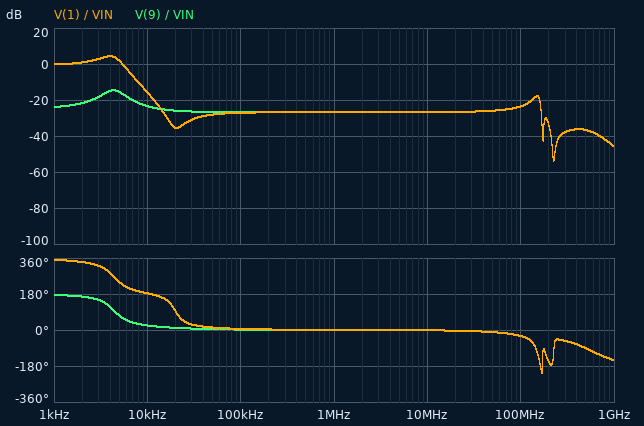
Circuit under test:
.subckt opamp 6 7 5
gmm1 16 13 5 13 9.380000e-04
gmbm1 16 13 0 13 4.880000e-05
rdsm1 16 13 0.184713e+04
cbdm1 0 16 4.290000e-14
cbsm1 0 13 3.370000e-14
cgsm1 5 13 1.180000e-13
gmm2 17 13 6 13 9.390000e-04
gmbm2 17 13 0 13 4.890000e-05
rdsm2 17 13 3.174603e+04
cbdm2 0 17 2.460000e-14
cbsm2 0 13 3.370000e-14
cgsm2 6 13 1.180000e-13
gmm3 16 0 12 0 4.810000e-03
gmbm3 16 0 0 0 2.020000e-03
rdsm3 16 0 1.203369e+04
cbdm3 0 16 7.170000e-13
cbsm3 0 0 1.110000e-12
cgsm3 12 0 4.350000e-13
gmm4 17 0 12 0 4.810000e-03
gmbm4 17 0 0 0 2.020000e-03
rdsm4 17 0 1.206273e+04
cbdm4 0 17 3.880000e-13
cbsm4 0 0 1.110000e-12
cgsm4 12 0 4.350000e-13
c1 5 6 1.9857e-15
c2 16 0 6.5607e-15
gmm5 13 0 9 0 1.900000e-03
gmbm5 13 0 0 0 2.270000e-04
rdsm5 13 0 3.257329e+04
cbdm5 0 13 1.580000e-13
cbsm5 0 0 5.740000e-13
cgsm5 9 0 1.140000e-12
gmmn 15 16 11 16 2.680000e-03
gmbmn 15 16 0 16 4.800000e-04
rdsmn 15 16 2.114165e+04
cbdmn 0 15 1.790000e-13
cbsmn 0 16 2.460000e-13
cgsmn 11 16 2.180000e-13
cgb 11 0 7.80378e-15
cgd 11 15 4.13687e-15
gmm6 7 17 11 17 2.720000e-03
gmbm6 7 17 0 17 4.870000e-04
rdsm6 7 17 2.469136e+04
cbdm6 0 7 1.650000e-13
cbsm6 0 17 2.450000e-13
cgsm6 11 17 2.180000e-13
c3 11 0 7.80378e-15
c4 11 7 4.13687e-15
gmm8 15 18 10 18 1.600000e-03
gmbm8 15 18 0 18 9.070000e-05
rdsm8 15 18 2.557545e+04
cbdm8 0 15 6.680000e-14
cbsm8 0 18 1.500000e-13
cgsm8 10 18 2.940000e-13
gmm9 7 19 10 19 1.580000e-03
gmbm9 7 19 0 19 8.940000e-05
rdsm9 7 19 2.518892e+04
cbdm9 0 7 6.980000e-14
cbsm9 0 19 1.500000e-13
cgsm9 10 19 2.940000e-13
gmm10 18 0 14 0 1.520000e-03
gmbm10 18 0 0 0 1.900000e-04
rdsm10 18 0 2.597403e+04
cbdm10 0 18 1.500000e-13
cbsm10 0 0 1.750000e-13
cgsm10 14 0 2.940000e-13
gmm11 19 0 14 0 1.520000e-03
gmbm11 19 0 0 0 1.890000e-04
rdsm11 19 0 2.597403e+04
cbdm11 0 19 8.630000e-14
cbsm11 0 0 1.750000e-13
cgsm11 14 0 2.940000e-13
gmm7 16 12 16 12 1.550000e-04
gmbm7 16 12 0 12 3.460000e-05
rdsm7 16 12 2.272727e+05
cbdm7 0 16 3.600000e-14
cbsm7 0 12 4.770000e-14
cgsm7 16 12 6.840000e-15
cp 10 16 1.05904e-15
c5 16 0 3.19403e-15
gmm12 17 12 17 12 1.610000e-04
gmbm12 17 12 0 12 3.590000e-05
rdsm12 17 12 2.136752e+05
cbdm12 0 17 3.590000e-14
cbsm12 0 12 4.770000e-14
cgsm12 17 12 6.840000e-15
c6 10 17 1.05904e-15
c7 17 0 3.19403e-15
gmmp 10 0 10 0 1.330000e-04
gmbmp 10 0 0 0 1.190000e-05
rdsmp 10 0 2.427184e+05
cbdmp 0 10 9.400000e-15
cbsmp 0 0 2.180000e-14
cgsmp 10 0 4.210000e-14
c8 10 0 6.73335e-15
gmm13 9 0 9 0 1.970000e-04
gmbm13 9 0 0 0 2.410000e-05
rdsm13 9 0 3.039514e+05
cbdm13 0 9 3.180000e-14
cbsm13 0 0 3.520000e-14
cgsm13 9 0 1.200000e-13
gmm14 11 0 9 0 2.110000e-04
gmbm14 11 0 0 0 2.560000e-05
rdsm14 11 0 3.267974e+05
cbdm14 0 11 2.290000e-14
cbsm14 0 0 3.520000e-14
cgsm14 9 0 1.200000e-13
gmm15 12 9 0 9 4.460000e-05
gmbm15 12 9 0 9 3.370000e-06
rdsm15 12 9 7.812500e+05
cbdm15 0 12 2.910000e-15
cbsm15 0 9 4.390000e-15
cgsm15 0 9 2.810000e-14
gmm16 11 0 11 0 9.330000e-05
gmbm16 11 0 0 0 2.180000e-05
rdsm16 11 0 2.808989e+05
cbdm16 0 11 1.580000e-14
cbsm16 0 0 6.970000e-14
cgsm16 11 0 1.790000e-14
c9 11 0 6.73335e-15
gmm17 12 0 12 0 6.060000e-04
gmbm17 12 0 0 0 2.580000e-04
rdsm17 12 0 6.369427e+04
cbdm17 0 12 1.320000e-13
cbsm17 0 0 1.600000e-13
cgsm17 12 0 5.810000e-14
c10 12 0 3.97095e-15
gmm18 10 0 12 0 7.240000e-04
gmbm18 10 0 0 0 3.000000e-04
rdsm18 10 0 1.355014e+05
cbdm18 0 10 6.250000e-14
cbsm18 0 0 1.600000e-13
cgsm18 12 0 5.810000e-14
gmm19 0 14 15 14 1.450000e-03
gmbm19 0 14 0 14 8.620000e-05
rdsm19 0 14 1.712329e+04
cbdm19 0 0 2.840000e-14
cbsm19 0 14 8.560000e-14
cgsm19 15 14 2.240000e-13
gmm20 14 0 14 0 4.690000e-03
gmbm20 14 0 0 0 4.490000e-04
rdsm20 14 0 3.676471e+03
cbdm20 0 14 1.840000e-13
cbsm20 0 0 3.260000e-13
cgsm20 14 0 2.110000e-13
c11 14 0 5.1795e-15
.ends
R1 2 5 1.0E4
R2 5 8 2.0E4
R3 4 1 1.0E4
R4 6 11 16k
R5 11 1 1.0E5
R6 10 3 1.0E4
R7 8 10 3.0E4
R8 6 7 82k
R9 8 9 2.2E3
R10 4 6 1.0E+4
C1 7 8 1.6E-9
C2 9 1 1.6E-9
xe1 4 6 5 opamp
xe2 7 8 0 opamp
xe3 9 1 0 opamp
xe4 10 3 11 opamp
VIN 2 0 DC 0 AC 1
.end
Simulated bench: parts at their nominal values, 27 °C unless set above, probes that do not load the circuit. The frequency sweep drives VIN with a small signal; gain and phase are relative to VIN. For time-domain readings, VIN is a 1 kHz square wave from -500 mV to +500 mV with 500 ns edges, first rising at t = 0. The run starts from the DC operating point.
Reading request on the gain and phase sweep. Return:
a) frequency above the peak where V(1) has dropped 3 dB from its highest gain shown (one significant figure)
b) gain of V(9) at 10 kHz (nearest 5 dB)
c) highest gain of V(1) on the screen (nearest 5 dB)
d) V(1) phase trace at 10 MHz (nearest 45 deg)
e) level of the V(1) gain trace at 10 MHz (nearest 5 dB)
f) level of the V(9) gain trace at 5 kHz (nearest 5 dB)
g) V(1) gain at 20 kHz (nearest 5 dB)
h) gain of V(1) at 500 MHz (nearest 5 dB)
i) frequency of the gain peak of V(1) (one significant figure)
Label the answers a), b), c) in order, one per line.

a) 5 kHz
b) -25 dB
c) 5 dB
d) 0 deg
e) -25 dB
f) -15 dB
g) -35 dB
h) -35 dB
i) 4 kHz
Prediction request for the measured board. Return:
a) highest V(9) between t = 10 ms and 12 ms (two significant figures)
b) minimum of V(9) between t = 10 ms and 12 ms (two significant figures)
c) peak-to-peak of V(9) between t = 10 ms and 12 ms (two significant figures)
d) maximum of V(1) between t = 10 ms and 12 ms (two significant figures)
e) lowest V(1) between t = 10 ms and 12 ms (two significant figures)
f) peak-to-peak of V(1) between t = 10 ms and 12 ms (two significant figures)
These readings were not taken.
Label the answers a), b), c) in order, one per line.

a) 73 mV
b) -73 mV
c) 150 mV
d) 810 mV
e) -810 mV
f) 1.6 V
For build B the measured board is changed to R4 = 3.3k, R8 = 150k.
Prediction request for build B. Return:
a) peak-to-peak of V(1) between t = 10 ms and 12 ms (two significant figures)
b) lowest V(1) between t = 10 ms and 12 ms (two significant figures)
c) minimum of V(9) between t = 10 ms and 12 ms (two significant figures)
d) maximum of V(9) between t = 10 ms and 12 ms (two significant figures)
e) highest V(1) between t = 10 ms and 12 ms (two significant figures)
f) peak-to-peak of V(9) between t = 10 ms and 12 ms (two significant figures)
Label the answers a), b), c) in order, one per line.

a) 1.5 V
b) -740 mV
c) -79 mV
d) 79 mV
e) 740 mV
f) 160 mV
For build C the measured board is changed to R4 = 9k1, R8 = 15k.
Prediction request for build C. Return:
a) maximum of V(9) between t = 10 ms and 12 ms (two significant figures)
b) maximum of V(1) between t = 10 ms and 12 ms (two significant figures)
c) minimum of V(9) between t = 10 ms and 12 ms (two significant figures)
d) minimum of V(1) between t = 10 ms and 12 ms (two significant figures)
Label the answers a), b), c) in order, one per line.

a) 110 mV
b) 980 mV
c) -110 mV
d) -980 mV
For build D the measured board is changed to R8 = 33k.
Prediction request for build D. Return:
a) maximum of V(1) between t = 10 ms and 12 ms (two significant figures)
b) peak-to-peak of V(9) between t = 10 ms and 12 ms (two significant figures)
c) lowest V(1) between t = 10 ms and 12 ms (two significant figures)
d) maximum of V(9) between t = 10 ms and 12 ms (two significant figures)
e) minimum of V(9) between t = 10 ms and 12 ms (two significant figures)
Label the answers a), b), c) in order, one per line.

a) 920 mV
b) 190 mV
c) -920 mV
d) 93 mV
e) -93 mV
